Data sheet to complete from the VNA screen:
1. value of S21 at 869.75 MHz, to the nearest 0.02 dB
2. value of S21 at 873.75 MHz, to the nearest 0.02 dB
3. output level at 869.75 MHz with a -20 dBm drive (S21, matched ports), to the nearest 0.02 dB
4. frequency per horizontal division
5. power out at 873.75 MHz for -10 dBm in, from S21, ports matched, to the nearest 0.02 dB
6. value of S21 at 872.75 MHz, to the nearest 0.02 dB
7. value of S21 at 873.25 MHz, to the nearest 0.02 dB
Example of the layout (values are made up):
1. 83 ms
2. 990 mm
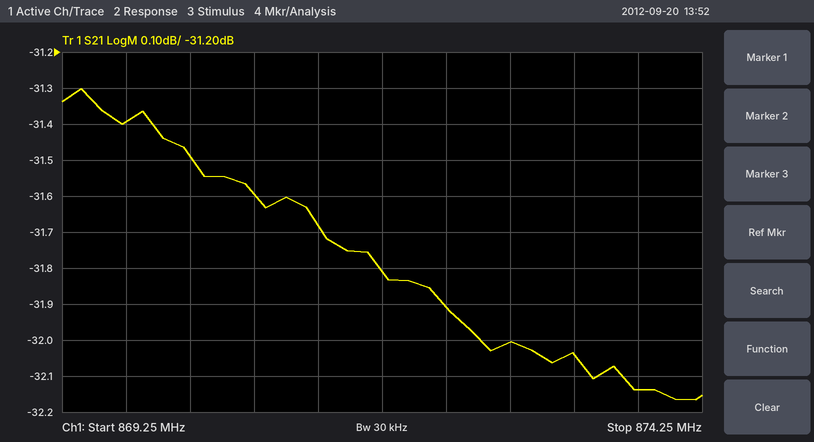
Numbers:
1. -31.40 dB
2. -32.14 dB
3. -51.40 dBm
4. 500 kHz
5. -42.14 dBm
6. -32.00 dB
7. -32.04 dB
